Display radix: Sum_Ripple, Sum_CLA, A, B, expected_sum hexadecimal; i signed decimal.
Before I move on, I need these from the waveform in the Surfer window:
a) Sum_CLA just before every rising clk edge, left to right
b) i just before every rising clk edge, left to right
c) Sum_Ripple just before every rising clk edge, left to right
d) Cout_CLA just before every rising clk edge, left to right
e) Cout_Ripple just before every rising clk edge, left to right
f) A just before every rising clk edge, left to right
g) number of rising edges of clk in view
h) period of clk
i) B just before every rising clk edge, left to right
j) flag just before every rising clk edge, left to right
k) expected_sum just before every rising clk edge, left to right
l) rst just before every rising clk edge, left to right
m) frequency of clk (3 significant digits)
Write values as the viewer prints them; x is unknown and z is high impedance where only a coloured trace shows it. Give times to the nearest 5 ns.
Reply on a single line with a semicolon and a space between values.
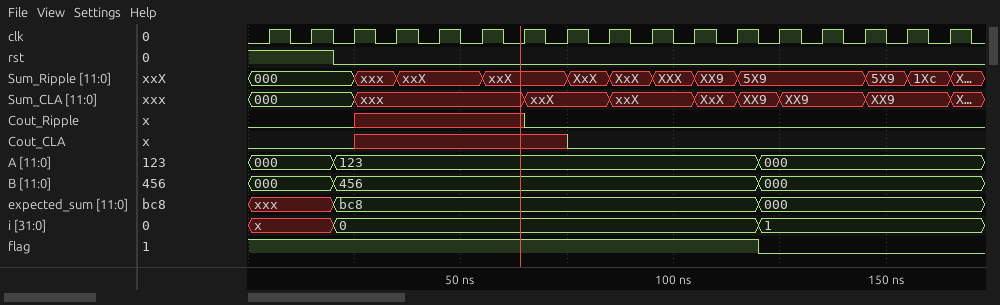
000, 000, 000, xxx, xxx, xxx, xxx, xxX, xxX, xxX, xxX, XxX, XX9, XX9, XX9, XX9, XX9; x, x, 0, 0, 0, 0, 0, 0, 0, 0, 0, 0, 1, 1, 1, 1, 1; 000, 000, 000, xxx, xxX, xxX, xxX, xxX, XxX, XxX, XXX, XX9, 5X9, 5X9, 5X9, 5X9, 1Xc; 0 0 0 x x x x x 0 0 0 0 0 0 0 0 0; 0 0 0 x x x x 0 0 0 0 0 0 0 0 0 0; 000, 000, 123, 123, 123, 123, 123, 123, 123, 123, 123, 123, 000, 000, 000, 000, 000; 17; 10 ns; 000, 000, 456, 456, 456, 456, 456, 456, 456, 456, 456, 456, 000, 000, 000, 000, 000; 1 1 1 1 1 1 1 1 1 1 1 1 0 0 0 0 0; xxx, xxx, bc8, bc8, bc8, bc8, bc8, bc8, bc8, bc8, bc8, bc8, 000, 000, 000, 000, 000; 1 1 0 0 0 0 0 0 0 0 0 0 0 0 0 0 0; 100 MHz
